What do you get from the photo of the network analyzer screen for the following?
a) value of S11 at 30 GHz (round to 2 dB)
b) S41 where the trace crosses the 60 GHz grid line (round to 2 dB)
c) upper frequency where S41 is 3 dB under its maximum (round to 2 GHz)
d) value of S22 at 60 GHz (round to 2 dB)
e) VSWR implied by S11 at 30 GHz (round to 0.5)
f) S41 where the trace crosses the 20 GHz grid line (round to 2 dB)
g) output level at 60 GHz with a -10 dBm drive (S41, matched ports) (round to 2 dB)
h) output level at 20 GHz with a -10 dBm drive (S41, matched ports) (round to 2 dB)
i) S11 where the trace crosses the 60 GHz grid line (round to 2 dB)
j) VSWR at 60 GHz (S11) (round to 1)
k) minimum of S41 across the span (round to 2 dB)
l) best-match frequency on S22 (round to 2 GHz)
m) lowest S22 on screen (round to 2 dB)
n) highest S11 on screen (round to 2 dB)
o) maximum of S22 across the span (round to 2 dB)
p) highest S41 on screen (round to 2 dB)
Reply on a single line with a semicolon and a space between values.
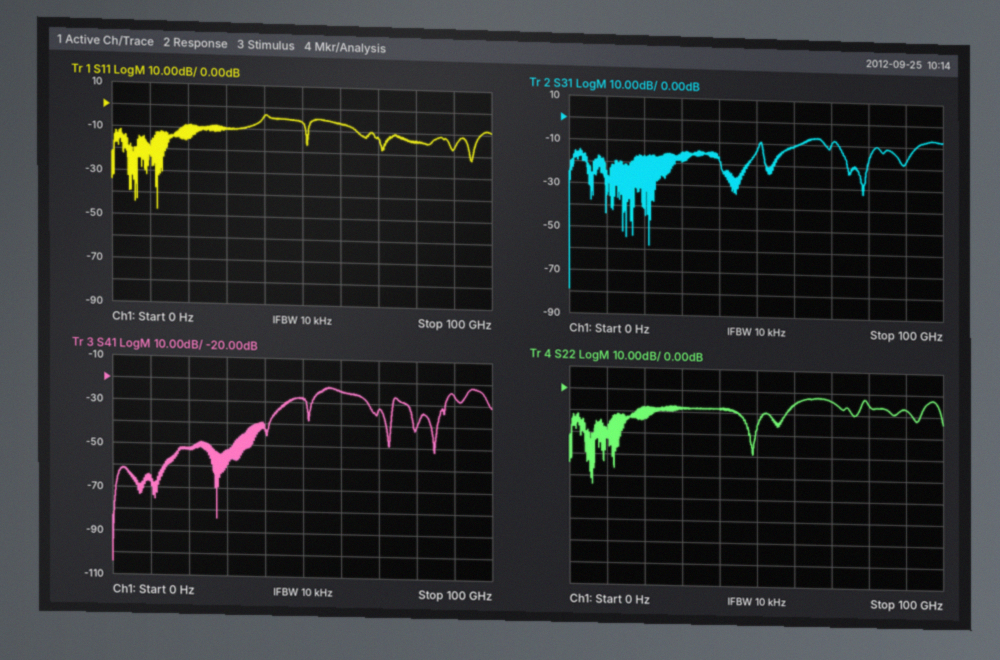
-10 dB; -24 dB; 98 GHz; -6 dB; 2.0; -52 dB; -34 dBm; -62 dBm; -6 dB; 3; -104 dB; 6 GHz; -44 dB; -4 dB; -2 dB; -22 dB
